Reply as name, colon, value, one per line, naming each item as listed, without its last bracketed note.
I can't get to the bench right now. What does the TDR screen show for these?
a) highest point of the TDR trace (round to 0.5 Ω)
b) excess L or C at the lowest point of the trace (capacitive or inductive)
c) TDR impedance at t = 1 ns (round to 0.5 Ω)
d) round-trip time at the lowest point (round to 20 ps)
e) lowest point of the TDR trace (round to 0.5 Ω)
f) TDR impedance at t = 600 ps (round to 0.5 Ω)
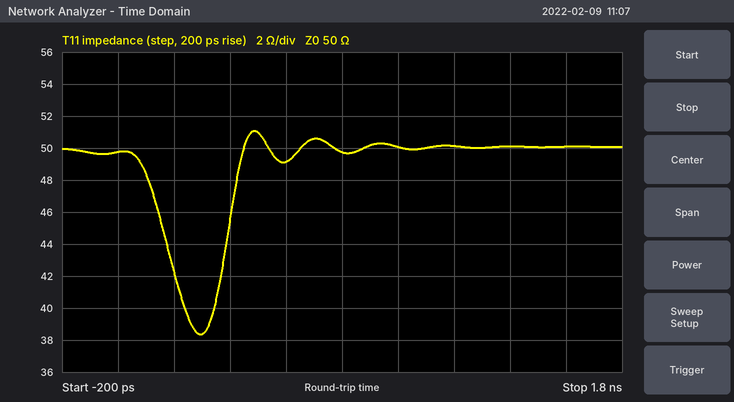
highest point of the TDR trace: 51.0 Ω
excess L or C at the lowest point of the trace: capacitive
TDR impedance at t = 1 ns: 50.0 Ω
round-trip time at the lowest point: 300 ps
lowest point of the TDR trace: 38.5 Ω
TDR impedance at t = 600 ps: 49.0 Ω
